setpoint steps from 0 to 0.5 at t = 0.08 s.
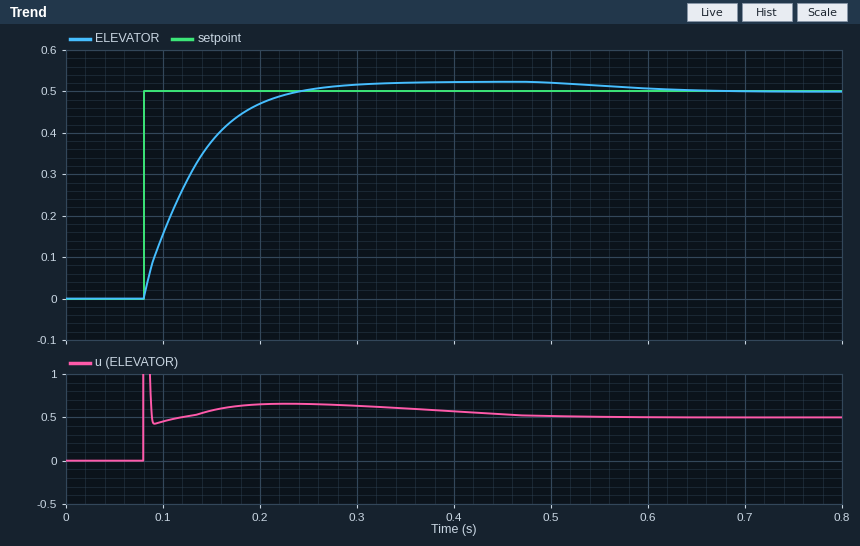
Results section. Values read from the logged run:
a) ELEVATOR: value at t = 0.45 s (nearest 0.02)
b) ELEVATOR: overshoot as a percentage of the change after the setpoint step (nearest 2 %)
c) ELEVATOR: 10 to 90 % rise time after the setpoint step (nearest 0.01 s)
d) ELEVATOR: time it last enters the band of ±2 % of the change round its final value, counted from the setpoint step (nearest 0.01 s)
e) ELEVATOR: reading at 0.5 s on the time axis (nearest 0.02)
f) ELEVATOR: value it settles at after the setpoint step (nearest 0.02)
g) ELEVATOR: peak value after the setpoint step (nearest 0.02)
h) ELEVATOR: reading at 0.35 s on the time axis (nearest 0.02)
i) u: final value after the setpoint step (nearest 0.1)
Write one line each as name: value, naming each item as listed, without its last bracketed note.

ELEVATOR: value at t = 0.45 s: 0.52
ELEVATOR: overshoot as a percentage of the change after the setpoint step: 4 %
ELEVATOR: 10 to 90 % rise time after the setpoint step: 0.10 s
ELEVATOR: time it last enters the band of ±2 % of the change round its final value, counted from the setpoint step: 0.50 s
ELEVATOR: reading at 0.5 s on the time axis: 0.52
ELEVATOR: value it settles at after the setpoint step: 0.50
ELEVATOR: peak value after the setpoint step: 0.52
ELEVATOR: reading at 0.35 s on the time axis: 0.52
u: final value after the setpoint step: 0.5
